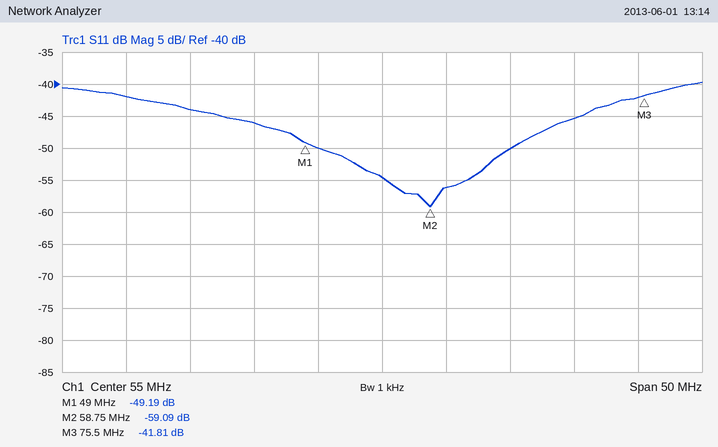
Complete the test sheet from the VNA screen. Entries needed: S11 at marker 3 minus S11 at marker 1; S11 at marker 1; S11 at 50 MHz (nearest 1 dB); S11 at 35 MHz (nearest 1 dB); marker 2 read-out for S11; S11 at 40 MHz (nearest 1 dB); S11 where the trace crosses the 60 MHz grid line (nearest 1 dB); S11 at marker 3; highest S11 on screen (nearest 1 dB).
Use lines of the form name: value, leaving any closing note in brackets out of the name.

S11 at marker 3 minus S11 at marker 1: 7.38 dB
S11 at marker 1: -49.19 dB
S11 at 50 MHz: -50 dB
S11 at 35 MHz: -42 dB
marker 2 read-out for S11: -59.09 dB
S11 at 40 MHz: -44 dB
S11 where the trace crosses the 60 MHz grid line: -56 dB
S11 at marker 3: -41.81 dB
highest S11 on screen: -40 dB
